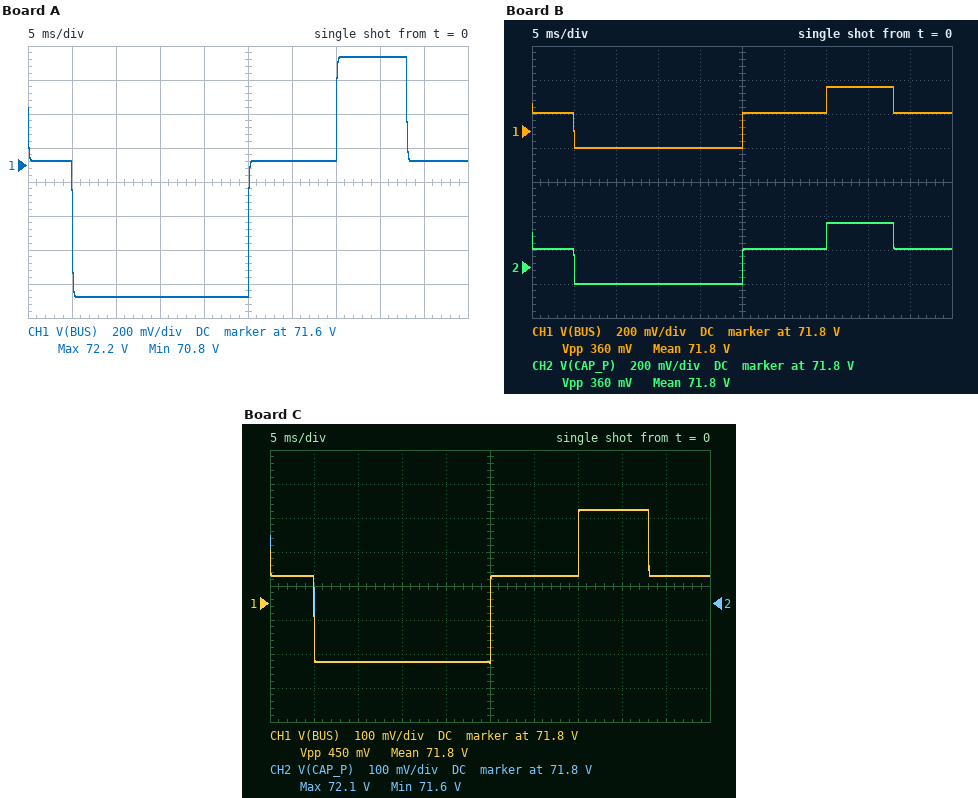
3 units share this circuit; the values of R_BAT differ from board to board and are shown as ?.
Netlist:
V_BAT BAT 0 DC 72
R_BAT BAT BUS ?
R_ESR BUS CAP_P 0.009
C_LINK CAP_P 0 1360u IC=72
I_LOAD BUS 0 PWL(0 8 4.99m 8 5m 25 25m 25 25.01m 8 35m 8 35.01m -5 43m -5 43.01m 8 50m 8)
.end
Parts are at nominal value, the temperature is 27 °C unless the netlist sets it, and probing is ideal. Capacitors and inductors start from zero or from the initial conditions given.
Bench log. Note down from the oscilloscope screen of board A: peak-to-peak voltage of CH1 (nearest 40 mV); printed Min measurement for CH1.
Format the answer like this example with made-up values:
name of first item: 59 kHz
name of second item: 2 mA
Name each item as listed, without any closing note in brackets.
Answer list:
peak-to-peak voltage of CH1: 1.40 V
printed Min measurement for CH1: 70.8 V
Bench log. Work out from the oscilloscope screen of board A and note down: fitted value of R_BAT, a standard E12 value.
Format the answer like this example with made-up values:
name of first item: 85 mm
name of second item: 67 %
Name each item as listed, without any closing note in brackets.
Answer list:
fitted value of R_BAT, a standard E12 value: 0.047 Ω
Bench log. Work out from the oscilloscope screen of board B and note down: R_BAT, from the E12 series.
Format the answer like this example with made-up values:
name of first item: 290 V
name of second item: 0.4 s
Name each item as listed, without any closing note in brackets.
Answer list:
R_BAT, from the E12 series: 0.012 Ω
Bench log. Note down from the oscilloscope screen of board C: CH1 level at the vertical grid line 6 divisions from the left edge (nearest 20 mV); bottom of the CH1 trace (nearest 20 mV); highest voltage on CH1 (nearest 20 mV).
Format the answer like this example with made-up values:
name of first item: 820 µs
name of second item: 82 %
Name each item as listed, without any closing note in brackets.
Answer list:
CH1 level at the vertical grid line 6 divisions from the left edge: 71.88 V
bottom of the CH1 trace: 71.62 V
highest voltage on CH1: 72.08 V
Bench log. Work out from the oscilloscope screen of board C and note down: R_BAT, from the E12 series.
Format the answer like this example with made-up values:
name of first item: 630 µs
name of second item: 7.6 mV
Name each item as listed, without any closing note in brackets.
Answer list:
R_BAT, from the E12 series: 0.015 Ω
